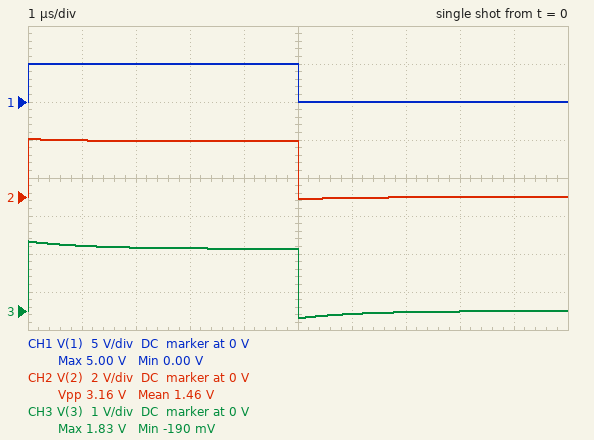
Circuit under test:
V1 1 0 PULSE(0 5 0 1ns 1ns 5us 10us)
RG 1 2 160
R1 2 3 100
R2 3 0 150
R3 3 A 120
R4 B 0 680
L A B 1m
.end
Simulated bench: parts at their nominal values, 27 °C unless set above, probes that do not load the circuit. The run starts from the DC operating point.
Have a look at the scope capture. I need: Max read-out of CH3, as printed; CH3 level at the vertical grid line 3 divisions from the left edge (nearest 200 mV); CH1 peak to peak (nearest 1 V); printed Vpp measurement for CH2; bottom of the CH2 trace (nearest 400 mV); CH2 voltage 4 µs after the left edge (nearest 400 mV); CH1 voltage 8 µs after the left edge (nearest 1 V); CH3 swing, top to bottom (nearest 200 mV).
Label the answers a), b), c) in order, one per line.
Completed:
a) 1.83 V
b) 1.6 V
c) 5 V
d) 3.16 V
e) 0 V
f) 2.8 V
g) 0 V
h) 2.0 V
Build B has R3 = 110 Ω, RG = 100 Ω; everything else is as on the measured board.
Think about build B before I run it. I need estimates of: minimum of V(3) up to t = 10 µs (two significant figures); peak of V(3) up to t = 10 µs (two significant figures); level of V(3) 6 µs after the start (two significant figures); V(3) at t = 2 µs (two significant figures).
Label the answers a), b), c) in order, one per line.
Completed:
a) -210 mV
b) 2.1 V
c) -86 mV
d) 2.0 V
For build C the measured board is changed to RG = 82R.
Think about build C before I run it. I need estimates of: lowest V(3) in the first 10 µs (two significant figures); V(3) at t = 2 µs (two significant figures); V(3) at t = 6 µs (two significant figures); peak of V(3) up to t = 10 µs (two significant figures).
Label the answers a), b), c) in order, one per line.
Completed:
a) -210 mV
b) 2.1 V
c) -86 mV
d) 2.3 V
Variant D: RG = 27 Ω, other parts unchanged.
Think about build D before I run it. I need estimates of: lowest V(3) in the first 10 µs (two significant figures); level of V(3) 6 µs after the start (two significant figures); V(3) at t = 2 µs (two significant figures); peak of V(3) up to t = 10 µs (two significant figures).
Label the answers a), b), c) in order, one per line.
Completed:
a) -210 mV
b) -89 mV
c) 2.5 V
d) 2.7 V
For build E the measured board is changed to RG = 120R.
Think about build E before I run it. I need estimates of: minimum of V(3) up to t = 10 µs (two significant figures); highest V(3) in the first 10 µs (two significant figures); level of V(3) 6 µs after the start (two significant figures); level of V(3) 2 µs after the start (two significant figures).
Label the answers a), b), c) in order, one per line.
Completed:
a) -200 mV
b) 2.0 V
c) -83 mV
d) 1.9 V
